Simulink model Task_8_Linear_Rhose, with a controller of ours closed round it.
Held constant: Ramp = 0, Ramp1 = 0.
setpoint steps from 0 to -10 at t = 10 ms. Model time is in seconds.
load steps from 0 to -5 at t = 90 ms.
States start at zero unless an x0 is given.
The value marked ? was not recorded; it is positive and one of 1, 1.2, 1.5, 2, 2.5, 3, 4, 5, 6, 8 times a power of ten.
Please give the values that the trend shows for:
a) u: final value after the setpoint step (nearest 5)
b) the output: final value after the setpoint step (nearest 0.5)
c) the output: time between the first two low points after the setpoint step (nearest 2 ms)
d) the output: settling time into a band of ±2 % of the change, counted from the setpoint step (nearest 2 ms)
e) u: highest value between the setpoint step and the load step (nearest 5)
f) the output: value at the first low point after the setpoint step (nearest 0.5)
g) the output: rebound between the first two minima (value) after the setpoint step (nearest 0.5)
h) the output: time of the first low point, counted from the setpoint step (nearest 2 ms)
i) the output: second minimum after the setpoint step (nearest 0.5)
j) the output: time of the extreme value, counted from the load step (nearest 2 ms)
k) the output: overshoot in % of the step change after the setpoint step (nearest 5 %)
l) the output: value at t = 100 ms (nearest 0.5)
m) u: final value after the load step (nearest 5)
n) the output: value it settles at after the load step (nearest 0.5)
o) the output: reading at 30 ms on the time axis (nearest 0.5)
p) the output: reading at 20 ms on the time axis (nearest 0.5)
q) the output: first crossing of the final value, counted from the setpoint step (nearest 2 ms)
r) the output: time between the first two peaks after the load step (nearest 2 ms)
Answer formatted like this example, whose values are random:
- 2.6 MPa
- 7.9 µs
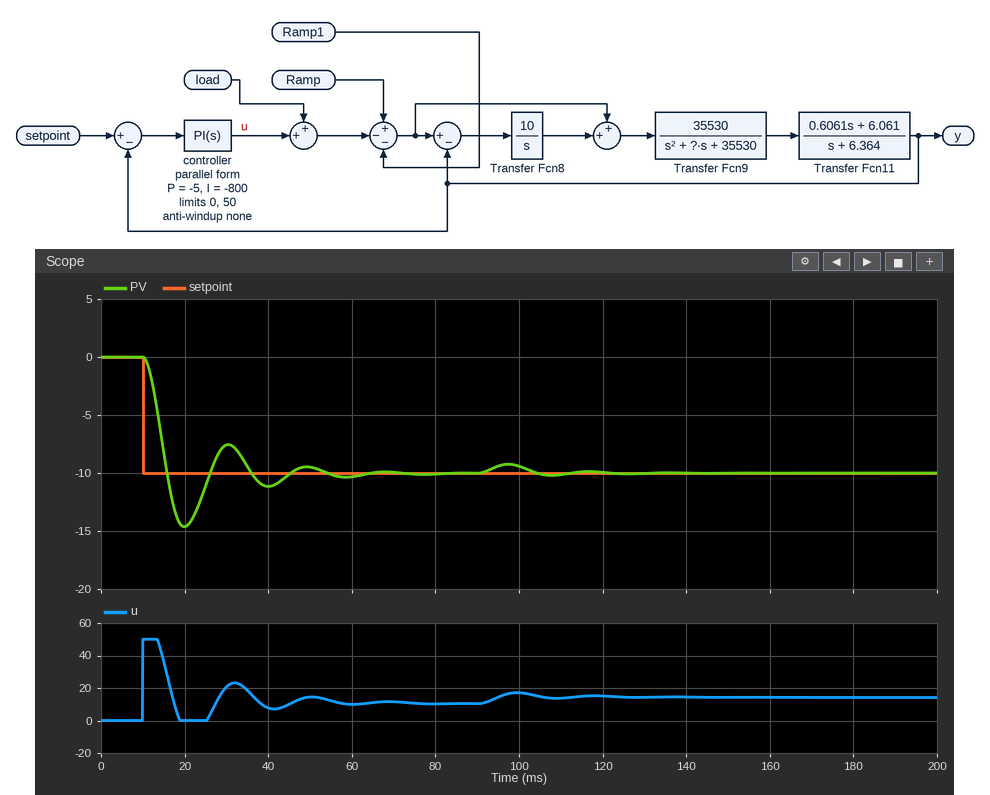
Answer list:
- 10
- -10.0
- 20 ms
- 52 ms
- 50
- -14.5
- -7.5
- 10 ms
- -11.0
- 8 ms
- 45 %
- -9.5
- 15
- -10.0
- -7.5
- -14.5
- 6 ms
- 20 ms
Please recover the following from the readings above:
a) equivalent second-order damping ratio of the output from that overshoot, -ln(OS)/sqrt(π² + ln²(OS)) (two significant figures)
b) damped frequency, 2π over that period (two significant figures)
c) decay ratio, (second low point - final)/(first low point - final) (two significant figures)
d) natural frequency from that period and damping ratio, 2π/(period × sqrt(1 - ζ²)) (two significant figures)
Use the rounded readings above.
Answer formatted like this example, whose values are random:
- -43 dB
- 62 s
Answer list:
- 0.25
- 0.31 rad/ms
- 0.22
- 0.32 rad/ms
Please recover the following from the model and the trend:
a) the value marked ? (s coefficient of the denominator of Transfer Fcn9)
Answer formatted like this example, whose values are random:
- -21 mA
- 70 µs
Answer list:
- 300
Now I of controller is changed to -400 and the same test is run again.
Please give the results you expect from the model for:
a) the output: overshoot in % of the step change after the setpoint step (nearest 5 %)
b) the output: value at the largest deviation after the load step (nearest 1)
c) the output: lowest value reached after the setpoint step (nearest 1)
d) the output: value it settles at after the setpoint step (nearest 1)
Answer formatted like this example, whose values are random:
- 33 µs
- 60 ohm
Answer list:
- 25 %
- -9
- -12
- -10
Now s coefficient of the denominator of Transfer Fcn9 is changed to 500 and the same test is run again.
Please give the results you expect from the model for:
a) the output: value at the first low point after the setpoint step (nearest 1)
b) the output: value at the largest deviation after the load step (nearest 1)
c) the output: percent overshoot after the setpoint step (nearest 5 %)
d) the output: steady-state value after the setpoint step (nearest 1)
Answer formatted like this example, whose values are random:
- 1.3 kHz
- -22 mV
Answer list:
- -13
- -9
- 35 %
- -10
